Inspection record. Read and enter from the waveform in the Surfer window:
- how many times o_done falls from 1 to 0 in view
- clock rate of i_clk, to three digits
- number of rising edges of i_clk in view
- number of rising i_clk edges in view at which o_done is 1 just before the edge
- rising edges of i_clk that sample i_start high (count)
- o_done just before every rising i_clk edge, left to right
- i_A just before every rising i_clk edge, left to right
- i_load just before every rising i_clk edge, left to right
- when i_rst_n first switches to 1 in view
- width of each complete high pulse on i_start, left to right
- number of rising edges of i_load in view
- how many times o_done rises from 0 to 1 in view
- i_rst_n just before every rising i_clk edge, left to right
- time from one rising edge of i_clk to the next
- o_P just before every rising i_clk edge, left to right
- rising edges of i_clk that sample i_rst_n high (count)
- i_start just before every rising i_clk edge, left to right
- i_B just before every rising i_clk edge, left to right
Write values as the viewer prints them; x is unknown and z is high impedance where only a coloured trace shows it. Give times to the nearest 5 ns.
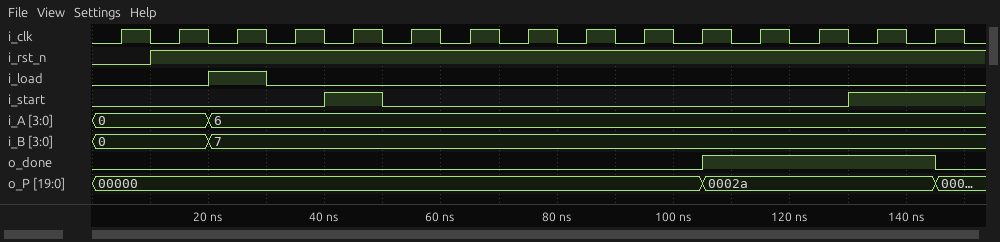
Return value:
1
100 MHz
15
4
3
0 0 0 0 0 0 0 0 0 0 0 1 1 1 1
0, 0, 6, 6, 6, 6, 6, 6, 6, 6, 6, 6, 6, 6, 6
0 0 1 0 0 0 0 0 0 0 0 0 0 0 0
10 ns
10 ns
1
1
0 1 1 1 1 1 1 1 1 1 1 1 1 1 1
10 ns
00000, 00000, 00000, 00000, 00000, 00000, 00000, 00000, 00000, 00000, 00000, 0002a, 0002a, 0002a, 0002a
14
0 0 0 0 1 0 0 0 0 0 0 0 0 1 1
0, 0, 7, 7, 7, 7, 7, 7, 7, 7, 7, 7, 7, 7, 7
